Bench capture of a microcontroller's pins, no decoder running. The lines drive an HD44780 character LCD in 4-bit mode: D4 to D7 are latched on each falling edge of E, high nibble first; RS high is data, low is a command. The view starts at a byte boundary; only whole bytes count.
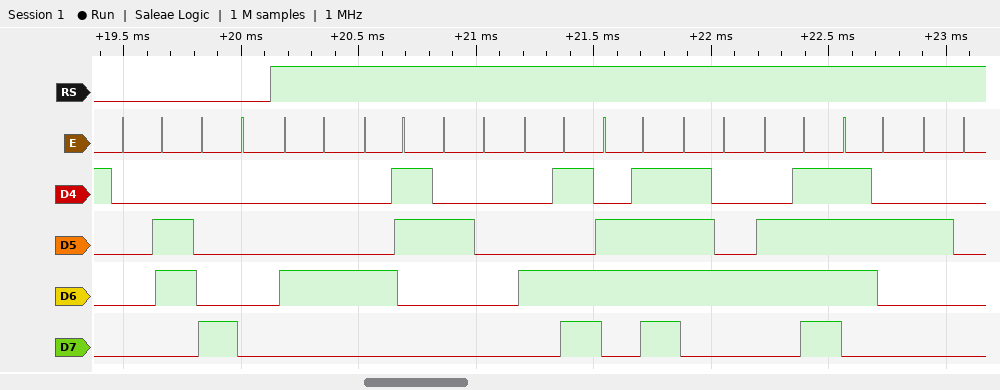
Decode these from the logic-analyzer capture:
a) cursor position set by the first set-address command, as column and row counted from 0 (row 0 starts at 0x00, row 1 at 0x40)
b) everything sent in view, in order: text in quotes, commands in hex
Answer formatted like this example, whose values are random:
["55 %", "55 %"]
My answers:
["column 0, row 0", "0x06 0x80 \"DC Motor \""]
